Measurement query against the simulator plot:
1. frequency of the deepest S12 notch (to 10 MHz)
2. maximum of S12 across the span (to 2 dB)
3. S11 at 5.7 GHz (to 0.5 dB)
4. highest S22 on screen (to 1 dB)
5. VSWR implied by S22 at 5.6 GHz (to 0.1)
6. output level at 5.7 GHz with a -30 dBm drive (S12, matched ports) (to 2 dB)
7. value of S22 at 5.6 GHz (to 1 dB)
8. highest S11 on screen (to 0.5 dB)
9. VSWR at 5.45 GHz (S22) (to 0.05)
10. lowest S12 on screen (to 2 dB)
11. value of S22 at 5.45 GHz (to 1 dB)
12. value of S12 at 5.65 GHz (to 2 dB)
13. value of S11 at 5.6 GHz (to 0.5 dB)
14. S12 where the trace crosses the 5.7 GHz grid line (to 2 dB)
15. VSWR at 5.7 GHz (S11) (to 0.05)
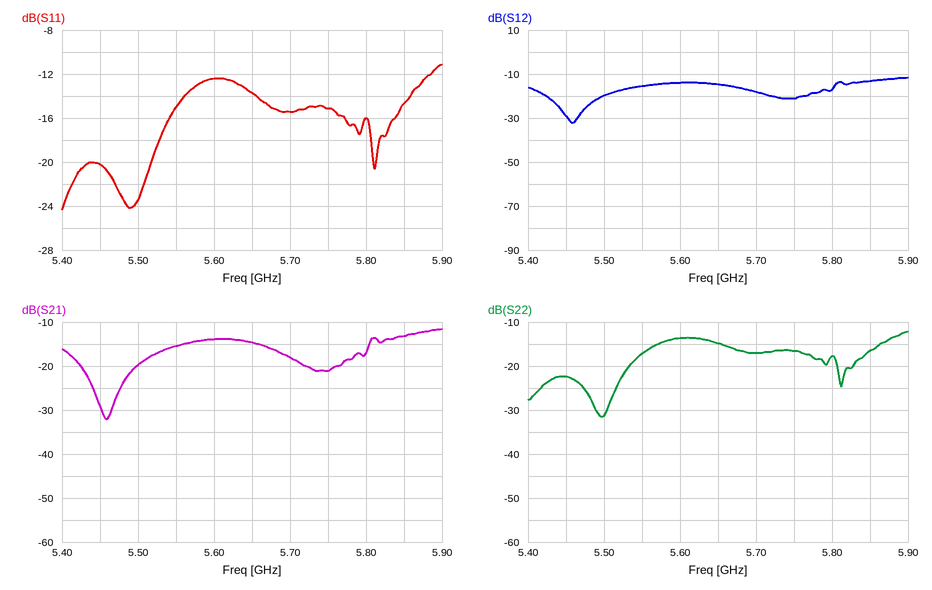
5.46 GHz
-12 dB
-15.5 dB
-12 dB
1.5
-48 dBm
-14 dB
-11.0 dB
1.15
-32 dB
-22 dB
-14 dB
-12.5 dB
-18 dB
1.40
